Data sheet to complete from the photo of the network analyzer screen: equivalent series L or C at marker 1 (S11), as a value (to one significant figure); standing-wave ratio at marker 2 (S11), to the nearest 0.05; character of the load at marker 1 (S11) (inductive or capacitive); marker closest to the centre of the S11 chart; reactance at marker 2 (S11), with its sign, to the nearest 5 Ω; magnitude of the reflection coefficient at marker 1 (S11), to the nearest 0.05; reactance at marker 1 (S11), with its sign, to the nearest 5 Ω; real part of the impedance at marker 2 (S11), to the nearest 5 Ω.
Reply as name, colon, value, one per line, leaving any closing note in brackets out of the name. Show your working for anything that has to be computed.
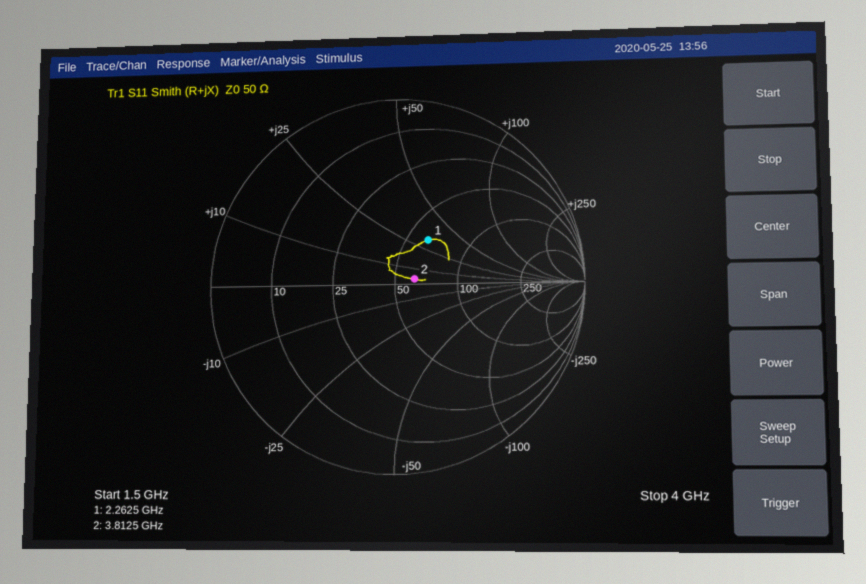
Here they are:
equivalent series L or C at marker 1 (S11), as a value: L = 30 Ω/(2π × 2.2625 GHz) ≈ 2 nH
standing-wave ratio at marker 2 (S11), to the nearest 0.05: 1.25
character of the load at marker 1 (S11): inductive
marker closest to the centre of the S11 chart: marker 2
reactance at marker 2 (S11), with its sign, to the nearest 5 Ω: +5 Ω
magnitude of the reflection coefficient at marker 1 (S11), to the nearest 0.05: 0.30
reactance at marker 1 (S11), with its sign, to the nearest 5 Ω: +30 Ω
real part of the impedance at marker 2 (S11), to the nearest 5 Ω: 60 Ω
